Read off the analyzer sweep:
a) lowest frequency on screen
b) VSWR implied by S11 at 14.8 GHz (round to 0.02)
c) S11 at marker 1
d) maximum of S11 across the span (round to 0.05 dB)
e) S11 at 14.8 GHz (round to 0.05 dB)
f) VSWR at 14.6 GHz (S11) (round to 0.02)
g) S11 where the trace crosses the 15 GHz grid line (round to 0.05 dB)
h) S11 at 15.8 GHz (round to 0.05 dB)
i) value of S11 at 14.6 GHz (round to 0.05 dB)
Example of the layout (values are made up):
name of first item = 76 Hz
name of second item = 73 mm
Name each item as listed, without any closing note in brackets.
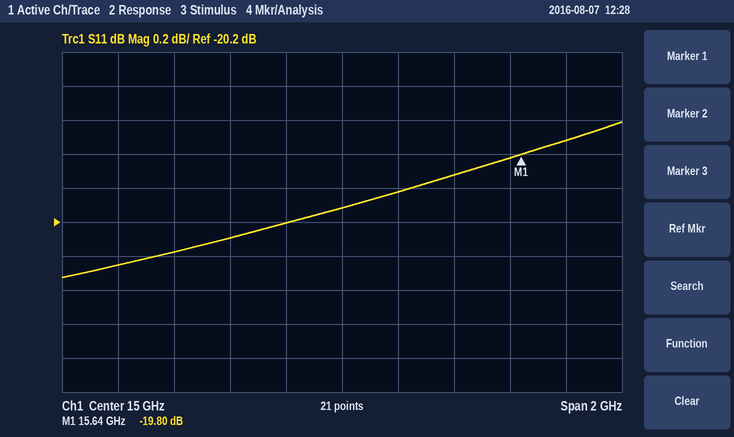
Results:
lowest frequency on screen = 14 GHz
VSWR implied by S11 at 14.8 GHz = 1.22
S11 at marker 1 = -19.80 dB
maximum of S11 across the span = -19.60 dB
S11 at 14.8 GHz = -20.20 dB
VSWR at 14.6 GHz (S11) = 1.22
S11 where the trace crosses the 15 GHz grid line = -20.10 dB
S11 at 15.8 GHz = -19.70 dB
value of S11 at 14.6 GHz = -20.30 dB
